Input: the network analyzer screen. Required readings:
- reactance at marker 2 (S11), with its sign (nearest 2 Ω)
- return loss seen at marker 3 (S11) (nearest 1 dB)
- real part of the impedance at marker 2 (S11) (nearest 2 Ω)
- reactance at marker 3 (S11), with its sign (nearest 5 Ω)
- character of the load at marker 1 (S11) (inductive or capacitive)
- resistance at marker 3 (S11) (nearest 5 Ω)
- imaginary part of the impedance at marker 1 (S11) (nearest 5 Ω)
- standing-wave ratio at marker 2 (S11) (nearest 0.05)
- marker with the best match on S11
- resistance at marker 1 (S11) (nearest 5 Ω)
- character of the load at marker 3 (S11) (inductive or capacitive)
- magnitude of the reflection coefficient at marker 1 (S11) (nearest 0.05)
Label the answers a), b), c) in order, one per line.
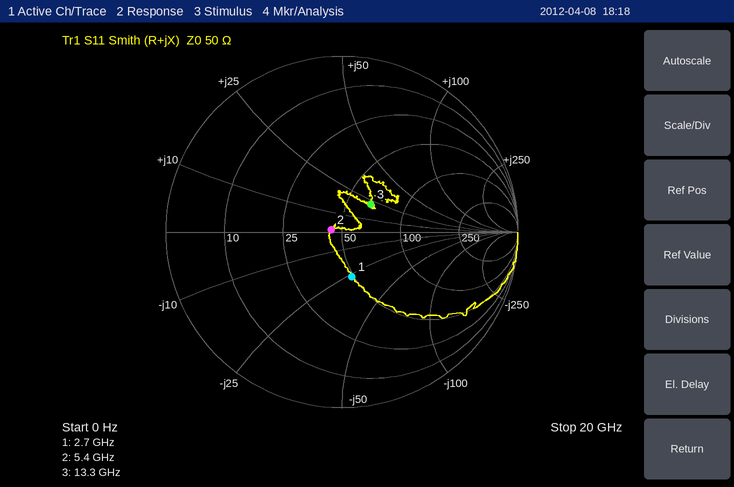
a) +2 Ω
b) 13 dB
c) 44 Ω
d) +20 Ω
e) capacitive
f) 65 Ω
g) -25 Ω
h) 1.15
i) marker 2
j) 50 Ω
k) inductive
l) 0.25
